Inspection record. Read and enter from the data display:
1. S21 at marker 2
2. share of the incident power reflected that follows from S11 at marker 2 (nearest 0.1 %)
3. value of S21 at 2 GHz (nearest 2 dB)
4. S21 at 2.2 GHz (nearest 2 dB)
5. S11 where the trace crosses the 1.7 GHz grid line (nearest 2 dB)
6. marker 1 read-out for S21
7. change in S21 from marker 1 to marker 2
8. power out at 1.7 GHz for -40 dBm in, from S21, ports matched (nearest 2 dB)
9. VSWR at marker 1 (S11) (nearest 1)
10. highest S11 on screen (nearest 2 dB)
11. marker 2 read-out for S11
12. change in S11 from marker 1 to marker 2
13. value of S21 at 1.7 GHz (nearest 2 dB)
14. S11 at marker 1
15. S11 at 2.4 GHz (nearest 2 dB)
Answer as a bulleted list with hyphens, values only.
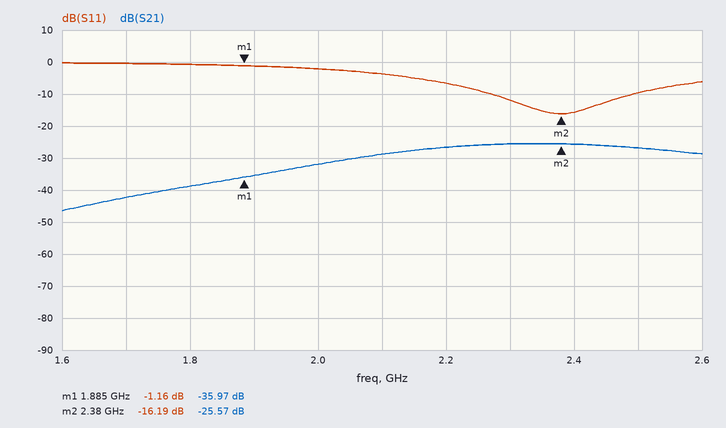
- -25.57 dB
- 2.4 %
- -32 dB
- -26 dB
- 0 dB
- -35.97 dB
- 10.40 dB
- -82 dBm
- 15
- 0 dB
- -16.19 dB
- -15.03 dB
- -42 dB
- -1.16 dB
- -16 dB
